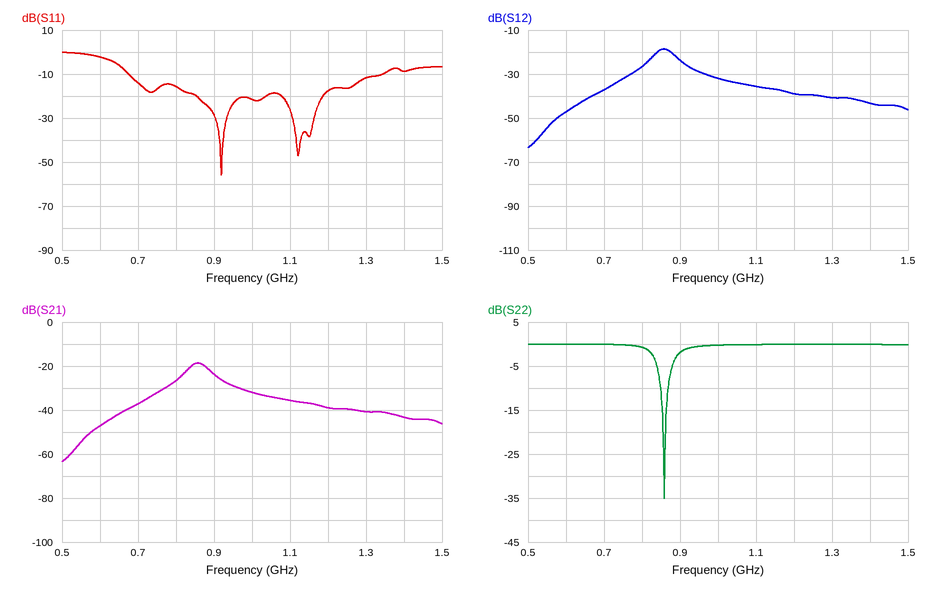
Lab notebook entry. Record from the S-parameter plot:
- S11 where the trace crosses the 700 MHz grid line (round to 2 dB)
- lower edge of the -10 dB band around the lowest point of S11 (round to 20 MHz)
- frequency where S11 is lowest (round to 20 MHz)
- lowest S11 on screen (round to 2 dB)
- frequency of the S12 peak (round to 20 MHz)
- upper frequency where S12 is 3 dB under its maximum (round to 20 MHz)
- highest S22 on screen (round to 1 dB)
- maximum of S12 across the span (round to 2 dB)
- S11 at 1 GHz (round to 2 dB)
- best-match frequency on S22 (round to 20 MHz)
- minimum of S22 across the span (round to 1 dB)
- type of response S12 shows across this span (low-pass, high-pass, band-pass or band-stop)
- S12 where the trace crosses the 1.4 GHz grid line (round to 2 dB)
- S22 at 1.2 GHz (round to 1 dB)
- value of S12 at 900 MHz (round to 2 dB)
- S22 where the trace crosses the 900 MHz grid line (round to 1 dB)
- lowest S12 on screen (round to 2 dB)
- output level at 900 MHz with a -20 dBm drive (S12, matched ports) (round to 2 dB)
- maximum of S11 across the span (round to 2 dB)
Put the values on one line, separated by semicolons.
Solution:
-14 dB; 680 MHz; 920 MHz; -56 dB; 860 MHz; 880 MHz; 0 dB; -18 dB; -22 dB; 860 MHz; -35 dB; band-pass; -44 dB; 0 dB; -24 dB; -2 dB; -64 dB; -44 dBm; 0 dB
